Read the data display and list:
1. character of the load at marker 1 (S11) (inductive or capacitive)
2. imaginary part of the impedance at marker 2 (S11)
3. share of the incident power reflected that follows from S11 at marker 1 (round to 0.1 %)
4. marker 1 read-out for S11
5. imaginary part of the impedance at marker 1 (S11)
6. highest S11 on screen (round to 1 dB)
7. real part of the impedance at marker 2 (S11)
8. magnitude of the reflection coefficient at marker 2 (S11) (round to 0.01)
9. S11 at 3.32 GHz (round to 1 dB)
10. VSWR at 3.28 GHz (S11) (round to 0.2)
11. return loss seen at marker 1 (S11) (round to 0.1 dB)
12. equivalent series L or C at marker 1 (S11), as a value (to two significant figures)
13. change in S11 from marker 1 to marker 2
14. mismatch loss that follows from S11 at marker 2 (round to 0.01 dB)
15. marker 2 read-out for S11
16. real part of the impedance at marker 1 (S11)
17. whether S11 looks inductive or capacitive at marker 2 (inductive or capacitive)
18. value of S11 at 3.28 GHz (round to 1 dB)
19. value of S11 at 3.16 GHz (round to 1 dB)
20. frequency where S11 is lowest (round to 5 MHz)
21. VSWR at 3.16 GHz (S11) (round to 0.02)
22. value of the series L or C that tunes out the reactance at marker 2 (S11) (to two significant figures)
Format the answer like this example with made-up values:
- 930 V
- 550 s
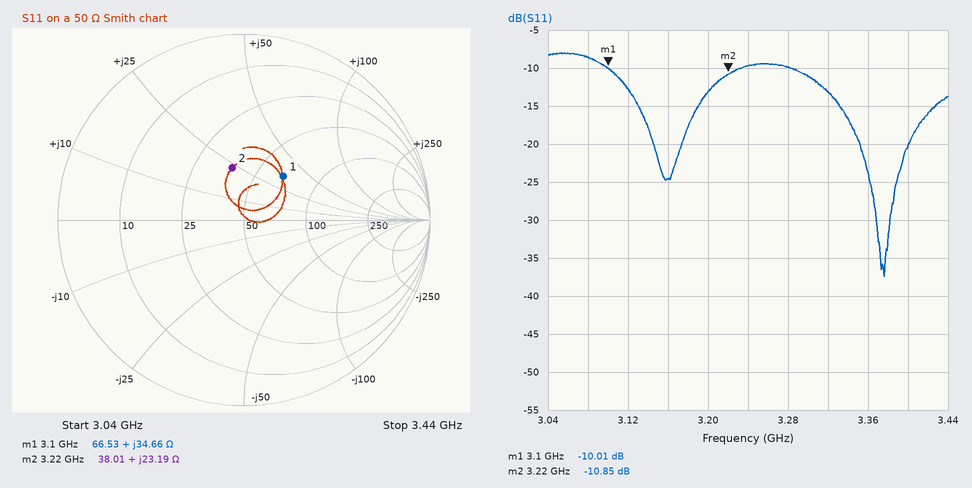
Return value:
- inductive
- +23.19 Ω
- 10.0 %
- -10.01 dB
- +34.66 Ω
- -8 dB
- 38.01 Ω
- 0.29
- -13 dB
- 2.0
- 10.0 dB
- 1.8 nH
- -0.84 dB
- 0.37 dB
- -10.85 dB
- 66.53 Ω
- inductive
- -10 dB
- -25 dB
- 3.375 GHz
- 1.12
- 2.1 pF
